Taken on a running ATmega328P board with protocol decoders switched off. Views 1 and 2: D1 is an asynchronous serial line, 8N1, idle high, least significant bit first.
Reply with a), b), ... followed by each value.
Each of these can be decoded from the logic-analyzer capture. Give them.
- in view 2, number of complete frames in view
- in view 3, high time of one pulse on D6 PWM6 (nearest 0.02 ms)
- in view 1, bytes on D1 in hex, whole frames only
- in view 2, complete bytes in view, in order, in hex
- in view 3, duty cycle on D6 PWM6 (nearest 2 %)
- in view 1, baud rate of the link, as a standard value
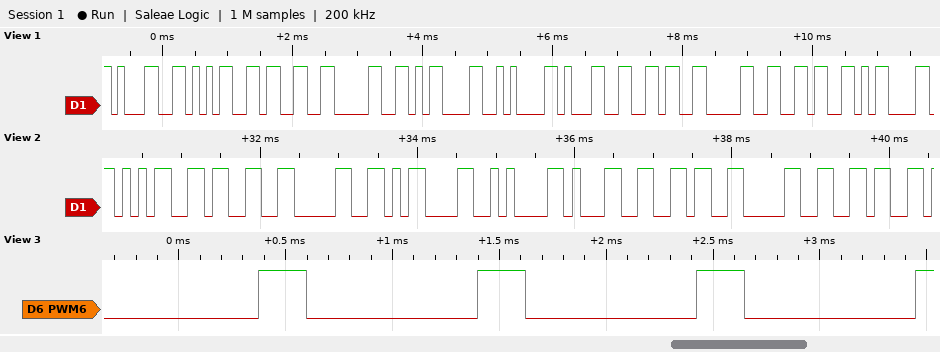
a) 9
b) 0.22 ms
c) 31 35 33 30 0D 0A 31 36 30 36 0D
d) 0x35 0x33 0x30 0x0D 0x0A 0x31 0x36 0x30 0x36
e) 22 %
f) 9600 baud
